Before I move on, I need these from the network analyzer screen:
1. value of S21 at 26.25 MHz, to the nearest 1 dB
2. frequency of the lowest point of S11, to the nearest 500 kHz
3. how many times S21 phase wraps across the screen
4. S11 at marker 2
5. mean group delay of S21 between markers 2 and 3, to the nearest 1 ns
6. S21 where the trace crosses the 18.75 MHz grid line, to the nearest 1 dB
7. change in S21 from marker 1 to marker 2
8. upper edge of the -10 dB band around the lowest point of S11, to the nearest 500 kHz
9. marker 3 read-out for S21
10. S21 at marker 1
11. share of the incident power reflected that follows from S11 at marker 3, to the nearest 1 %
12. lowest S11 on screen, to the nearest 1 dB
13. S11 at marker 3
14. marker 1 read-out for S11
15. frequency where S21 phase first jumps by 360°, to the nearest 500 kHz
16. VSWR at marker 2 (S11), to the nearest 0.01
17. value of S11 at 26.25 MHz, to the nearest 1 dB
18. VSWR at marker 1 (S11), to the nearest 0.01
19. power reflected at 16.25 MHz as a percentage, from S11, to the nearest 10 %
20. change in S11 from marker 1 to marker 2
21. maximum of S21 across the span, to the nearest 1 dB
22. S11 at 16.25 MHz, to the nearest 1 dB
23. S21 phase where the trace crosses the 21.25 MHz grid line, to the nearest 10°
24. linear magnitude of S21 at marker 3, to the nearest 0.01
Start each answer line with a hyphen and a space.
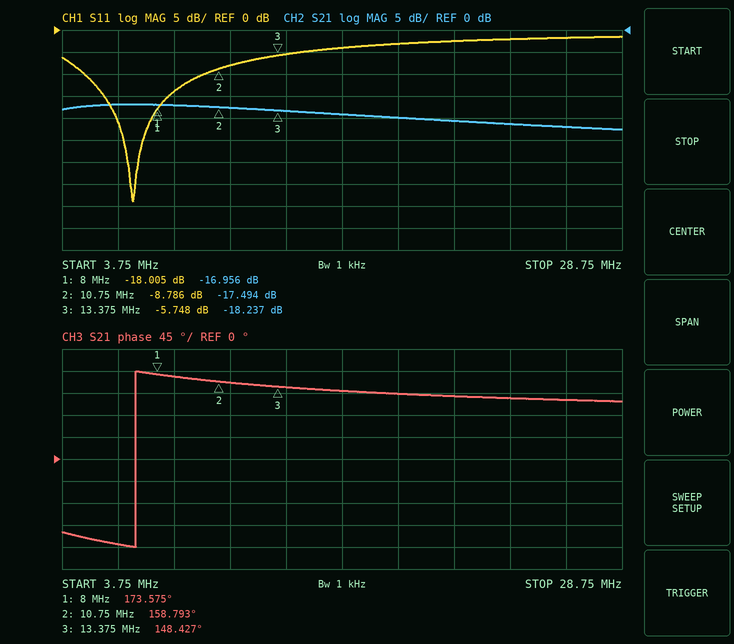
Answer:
- -22 dB
- 7.0 MHz
- 1
- -8.786 dB
- 11 ns
- -20 dB
- -0.538 dB
- 10.0 MHz
- -18.237 dB
- -16.956 dB
- 27 %
- -39 dB
- -5.748 dB
- -18.005 dB
- 7.0 MHz
- 2.14
- -2 dB
- 1.29
- 40 %
- 9.219 dB
- -17 dB
- -4 dB
- 130°
- 0.12
